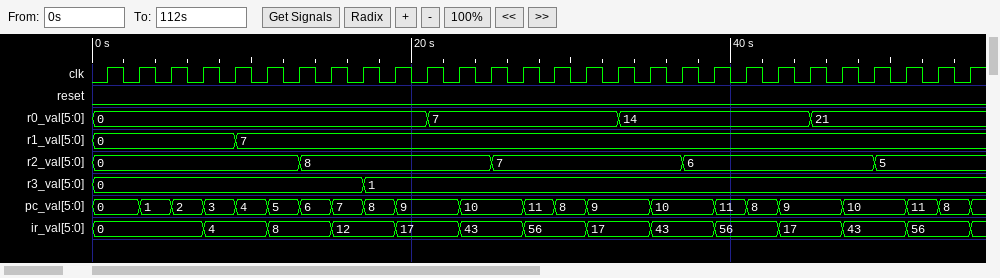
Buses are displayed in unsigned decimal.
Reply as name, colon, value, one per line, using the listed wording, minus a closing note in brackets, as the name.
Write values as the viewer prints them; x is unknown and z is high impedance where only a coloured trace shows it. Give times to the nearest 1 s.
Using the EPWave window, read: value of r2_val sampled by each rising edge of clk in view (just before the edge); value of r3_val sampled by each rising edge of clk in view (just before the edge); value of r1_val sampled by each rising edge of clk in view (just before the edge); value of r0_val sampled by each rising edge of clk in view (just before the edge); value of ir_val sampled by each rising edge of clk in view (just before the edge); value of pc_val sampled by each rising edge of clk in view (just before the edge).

value of r2_val sampled by each rising edge of clk in view: 0, 0, 0, 0, 0, 0, 0, 8, 8, 8, 8, 8, 8, 7, 7, 7, 7, 7, 7, 6, 6, 6, 6, 6, 6, 5, 5, 5
value of r3_val sampled by each rising edge of clk in view: 0, 0, 0, 0, 0, 0, 0, 0, 0, 1, 1, 1, 1, 1, 1, 1, 1, 1, 1, 1, 1, 1, 1, 1, 1, 1, 1, 1
value of r1_val sampled by each rising edge of clk in view: 0, 0, 0, 0, 0, 7, 7, 7, 7, 7, 7, 7, 7, 7, 7, 7, 7, 7, 7, 7, 7, 7, 7, 7, 7, 7, 7, 7
value of r0_val sampled by each rising edge of clk in view: 0, 0, 0, 0, 0, 0, 0, 0, 0, 0, 0, 7, 7, 7, 7, 7, 7, 14, 14, 14, 14, 14, 14, 21, 21, 21, 21, 21
value of ir_val sampled by each rising edge of clk in view: 0, 0, 0, 0, 4, 4, 8, 8, 12, 12, 17, 17, 43, 43, 56, 56, 17, 17, 43, 43, 56, 56, 17, 17, 43, 43, 56, 56
value of pc_val sampled by each rising edge of clk in view: 0, 0, 1, 2, 3, 4, 5, 6, 7, 8, 9, 9, 10, 10, 11, 8, 9, 9, 10, 10, 11, 8, 9, 9, 10, 10, 11, 8
